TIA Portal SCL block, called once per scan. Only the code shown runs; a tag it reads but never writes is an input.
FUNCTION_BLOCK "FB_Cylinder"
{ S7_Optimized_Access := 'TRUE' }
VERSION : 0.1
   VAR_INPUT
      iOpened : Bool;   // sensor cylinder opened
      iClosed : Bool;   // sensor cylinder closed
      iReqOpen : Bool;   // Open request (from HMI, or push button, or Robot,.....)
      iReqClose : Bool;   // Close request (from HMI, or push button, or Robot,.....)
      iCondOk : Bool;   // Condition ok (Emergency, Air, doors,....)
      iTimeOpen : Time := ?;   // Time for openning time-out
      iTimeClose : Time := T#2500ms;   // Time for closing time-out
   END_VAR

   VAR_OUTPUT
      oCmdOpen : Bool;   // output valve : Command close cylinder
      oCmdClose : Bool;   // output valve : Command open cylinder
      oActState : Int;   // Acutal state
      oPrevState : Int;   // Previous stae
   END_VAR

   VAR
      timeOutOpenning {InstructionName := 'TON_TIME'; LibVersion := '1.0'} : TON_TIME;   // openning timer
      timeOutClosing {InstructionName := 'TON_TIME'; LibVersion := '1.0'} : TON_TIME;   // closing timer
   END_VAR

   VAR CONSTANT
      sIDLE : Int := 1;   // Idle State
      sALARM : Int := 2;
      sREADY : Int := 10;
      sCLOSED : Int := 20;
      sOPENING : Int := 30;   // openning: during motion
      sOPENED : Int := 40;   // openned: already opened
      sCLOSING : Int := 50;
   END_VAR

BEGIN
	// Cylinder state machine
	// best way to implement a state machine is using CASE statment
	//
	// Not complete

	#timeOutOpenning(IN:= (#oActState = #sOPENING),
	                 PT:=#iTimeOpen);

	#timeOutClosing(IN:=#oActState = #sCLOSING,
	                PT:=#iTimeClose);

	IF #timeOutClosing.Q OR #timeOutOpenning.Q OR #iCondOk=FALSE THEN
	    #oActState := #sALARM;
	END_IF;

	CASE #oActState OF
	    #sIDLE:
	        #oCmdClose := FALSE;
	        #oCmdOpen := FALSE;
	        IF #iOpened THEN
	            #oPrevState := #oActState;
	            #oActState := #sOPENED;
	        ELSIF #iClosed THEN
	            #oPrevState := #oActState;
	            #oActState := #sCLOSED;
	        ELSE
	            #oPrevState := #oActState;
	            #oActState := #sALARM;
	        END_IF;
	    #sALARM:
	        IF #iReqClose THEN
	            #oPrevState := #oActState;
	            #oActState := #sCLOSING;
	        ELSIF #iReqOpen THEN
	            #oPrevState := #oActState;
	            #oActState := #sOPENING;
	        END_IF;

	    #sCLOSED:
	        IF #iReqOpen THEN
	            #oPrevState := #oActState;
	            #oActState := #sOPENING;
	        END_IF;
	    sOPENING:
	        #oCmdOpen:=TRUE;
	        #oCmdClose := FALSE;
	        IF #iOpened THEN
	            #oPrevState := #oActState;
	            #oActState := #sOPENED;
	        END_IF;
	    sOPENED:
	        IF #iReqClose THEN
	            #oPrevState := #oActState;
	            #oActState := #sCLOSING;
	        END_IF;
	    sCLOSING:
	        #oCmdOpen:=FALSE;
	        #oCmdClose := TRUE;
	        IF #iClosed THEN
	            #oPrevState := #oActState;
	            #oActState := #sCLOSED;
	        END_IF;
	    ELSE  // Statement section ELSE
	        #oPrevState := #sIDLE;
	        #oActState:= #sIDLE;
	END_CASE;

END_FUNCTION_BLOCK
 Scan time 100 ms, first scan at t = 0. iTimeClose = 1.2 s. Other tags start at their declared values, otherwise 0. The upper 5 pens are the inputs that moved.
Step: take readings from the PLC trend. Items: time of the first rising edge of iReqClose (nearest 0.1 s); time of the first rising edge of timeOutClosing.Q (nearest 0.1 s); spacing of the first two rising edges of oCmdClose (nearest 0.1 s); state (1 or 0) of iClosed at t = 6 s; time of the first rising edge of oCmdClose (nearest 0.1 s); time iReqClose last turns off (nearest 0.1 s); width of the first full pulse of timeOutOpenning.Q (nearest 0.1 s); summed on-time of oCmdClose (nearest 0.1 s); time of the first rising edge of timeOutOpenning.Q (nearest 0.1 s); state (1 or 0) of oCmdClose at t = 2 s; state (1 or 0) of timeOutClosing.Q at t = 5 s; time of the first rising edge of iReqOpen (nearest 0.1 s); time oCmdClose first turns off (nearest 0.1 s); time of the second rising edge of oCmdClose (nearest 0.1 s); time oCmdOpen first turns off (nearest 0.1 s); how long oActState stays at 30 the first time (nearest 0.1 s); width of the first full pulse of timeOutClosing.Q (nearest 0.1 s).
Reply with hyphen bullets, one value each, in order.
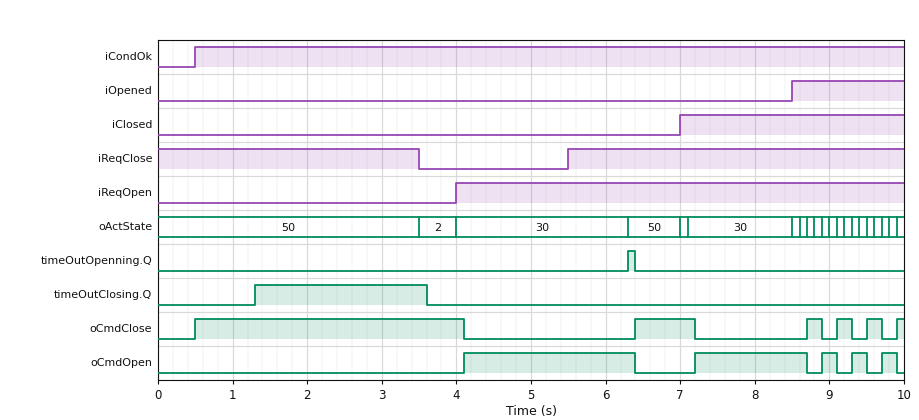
- 5.5 s
- 1.3 s
- 5.9 s
- 0
- 0.5 s
- 3.5 s
- 0.1 s
- 5.1 s
- 6.3 s
- 1
- 0
- 4.0 s
- 4.1 s
- 6.4 s
- 6.4 s
- 2.3 s
- 2.3 s
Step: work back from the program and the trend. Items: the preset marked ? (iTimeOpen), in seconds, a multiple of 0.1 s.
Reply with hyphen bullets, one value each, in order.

- 2.2 s
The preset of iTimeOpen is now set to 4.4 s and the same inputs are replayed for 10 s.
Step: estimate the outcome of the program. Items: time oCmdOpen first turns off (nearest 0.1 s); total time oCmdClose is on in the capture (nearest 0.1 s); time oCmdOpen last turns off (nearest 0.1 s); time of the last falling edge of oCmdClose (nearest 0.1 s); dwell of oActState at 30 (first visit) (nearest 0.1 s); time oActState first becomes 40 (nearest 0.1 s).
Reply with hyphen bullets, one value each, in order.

- 8.6 s
- 4.4 s
- 9.8 s
- 9.6 s
- 4.5 s
- 8.8 s
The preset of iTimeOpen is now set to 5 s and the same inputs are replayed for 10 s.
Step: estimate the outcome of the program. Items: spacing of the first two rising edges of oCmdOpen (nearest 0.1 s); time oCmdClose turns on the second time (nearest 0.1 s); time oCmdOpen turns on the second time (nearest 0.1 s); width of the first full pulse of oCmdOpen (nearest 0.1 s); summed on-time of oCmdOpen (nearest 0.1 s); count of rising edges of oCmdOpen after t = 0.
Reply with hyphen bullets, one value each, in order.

- 4.8 s
- 8.7 s
- 8.9 s
- 4.6 s
- 5.2 s
- 4
